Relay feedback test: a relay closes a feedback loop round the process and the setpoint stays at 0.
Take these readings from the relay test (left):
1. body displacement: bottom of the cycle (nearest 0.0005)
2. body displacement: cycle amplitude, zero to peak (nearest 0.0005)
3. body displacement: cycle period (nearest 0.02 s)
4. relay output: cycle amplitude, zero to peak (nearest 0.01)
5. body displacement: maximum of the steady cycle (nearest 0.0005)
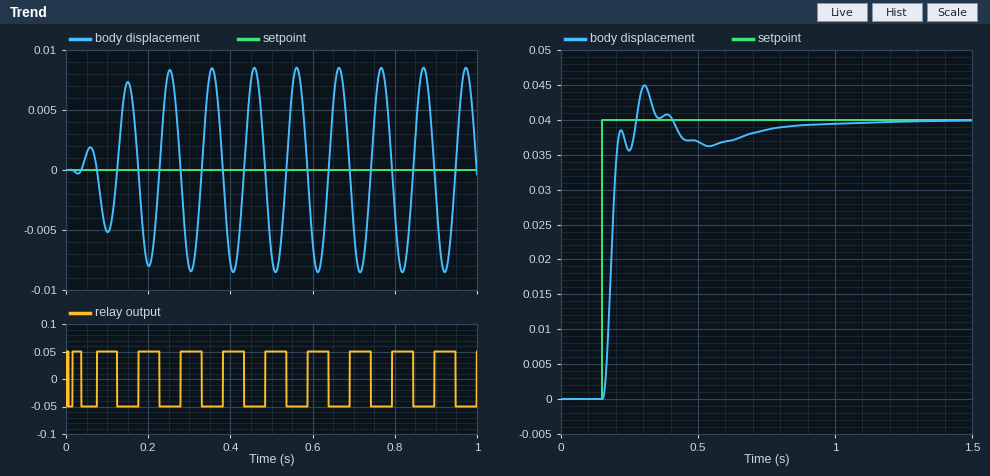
-0.0085
0.0085
0.10 s
0.05
0.0085
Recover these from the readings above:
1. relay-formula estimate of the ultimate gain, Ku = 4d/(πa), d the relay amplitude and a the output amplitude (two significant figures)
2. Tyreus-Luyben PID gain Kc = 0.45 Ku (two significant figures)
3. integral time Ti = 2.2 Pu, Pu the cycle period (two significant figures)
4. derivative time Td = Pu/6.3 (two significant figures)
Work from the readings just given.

7.5
3.4
0.22 s
0.016 s
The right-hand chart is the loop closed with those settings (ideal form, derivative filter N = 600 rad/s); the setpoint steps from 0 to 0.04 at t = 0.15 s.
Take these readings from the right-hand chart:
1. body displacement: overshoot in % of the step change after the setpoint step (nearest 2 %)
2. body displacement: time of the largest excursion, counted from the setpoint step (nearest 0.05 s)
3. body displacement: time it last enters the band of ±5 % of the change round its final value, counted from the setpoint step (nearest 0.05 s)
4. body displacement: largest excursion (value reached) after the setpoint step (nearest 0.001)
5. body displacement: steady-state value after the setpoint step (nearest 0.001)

12 %
0.15 s
0.55 s
0.045
0.040
